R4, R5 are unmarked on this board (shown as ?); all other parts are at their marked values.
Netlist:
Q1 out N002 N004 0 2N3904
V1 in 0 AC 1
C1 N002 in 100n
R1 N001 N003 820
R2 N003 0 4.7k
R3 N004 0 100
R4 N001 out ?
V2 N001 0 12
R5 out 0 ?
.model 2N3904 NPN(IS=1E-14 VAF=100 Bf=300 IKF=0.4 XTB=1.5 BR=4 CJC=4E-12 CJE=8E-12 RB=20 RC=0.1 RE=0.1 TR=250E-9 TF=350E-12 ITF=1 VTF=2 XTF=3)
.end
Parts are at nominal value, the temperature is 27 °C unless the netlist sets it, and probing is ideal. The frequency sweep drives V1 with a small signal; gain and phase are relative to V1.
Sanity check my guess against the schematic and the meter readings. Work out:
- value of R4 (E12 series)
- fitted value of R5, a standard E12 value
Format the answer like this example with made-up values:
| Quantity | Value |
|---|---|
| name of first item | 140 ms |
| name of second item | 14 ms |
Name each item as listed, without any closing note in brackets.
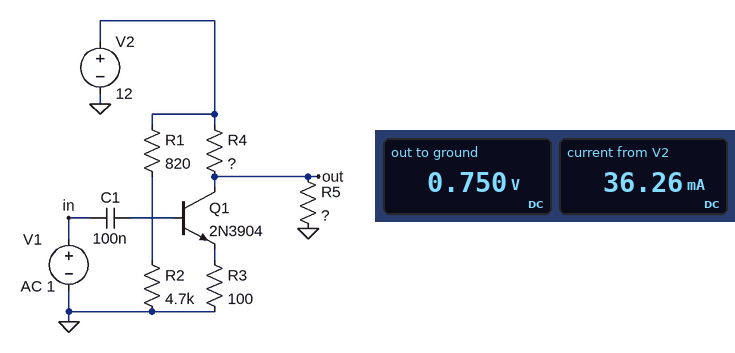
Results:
| Quantity | Value |
|---|---|
| value of R4 | 330 Ω |
| fitted value of R5, a standard E12 value | 22 Ω |
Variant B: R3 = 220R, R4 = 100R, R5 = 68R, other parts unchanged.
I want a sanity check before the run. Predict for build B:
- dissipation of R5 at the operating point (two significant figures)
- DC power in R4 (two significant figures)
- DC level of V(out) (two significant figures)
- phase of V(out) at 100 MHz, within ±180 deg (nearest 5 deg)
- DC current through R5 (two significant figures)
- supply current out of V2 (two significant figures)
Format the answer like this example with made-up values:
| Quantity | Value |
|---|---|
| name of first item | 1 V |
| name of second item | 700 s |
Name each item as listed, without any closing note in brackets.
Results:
| Quantity | Value |
|---|---|
| dissipation of R5 at the operating point | 350 mW |
| DC power in R4 | 510 mW |
| DC level of V(out) | 4.9 V |
| phase of V(out) at 100 MHz, within ±180 deg | 85 deg |
| DC current through R5 | 71 mA |
| supply current out of V2 | 74 mA |
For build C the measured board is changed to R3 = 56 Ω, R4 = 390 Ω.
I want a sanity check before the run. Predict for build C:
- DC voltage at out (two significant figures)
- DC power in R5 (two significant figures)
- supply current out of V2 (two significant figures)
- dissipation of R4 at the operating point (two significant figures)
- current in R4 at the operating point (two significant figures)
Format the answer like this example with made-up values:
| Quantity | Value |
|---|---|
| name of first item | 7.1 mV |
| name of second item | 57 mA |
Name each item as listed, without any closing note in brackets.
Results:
| Quantity | Value |
|---|---|
| DC voltage at out | 640 mV |
| DC power in R5 | 19 mW |
| supply current out of V2 | 31 mA |
| dissipation of R4 at the operating point | 330 mW |
| current in R4 at the operating point | 29 mA |
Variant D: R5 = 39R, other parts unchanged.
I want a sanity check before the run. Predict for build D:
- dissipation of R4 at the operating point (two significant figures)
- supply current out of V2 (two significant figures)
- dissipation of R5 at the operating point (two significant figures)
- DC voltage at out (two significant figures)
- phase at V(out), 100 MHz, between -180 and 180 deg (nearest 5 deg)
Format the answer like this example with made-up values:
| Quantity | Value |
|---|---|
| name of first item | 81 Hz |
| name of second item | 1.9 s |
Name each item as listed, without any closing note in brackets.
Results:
| Quantity | Value |
|---|---|
| dissipation of R4 at the operating point | 350 mW |
| supply current out of V2 | 35 mA |
| dissipation of R5 at the operating point | 41 mW |
| DC voltage at out | 1.3 V |
| phase at V(out), 100 MHz, between -180 and 180 deg | 80 deg |
